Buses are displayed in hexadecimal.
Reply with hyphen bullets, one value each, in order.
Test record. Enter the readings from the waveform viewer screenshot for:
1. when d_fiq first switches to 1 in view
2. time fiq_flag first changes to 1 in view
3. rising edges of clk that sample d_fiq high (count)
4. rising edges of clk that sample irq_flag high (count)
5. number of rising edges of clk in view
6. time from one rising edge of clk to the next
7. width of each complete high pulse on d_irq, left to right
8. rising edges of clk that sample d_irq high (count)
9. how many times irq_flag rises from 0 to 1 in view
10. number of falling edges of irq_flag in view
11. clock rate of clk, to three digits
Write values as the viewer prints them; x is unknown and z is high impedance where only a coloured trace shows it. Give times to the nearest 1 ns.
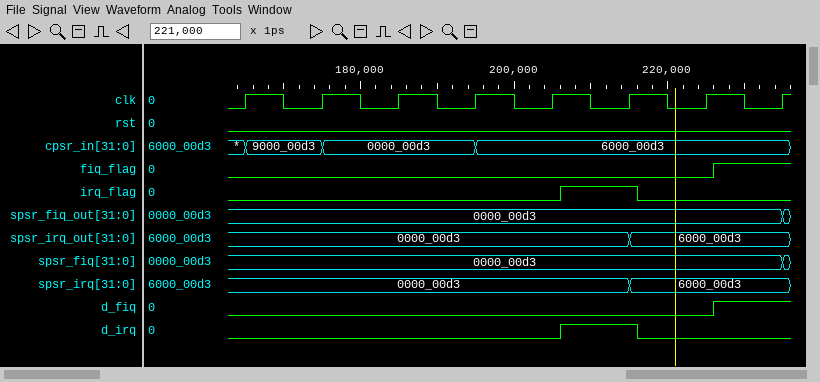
- 226 ns
- 226 ns
- 1
- 1
- 8
- 10 ns
- 10 ns
- 1
- 1
- 1
- 100 MHz
